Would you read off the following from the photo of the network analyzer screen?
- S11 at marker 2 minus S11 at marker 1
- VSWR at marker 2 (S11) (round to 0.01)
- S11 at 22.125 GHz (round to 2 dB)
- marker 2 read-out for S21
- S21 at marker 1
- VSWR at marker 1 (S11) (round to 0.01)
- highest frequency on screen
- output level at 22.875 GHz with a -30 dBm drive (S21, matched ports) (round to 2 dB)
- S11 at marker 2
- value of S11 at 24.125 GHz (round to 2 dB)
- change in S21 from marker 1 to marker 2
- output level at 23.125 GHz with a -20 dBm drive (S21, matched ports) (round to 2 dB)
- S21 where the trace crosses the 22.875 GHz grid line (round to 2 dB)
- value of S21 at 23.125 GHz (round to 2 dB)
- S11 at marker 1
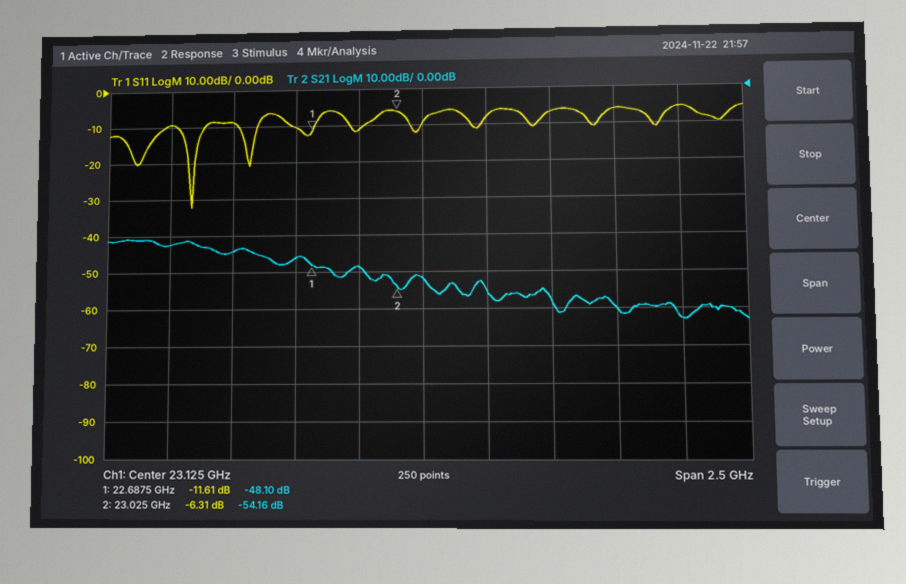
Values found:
5.30 dB
2.87
-10 dB
-54.16 dB
-48.10 dB
1.71
24.375 GHz
-78 dBm
-6.31 dB
-6 dB
-6.06 dB
-72 dBm
-48 dB
-52 dB
-11.61 dB
